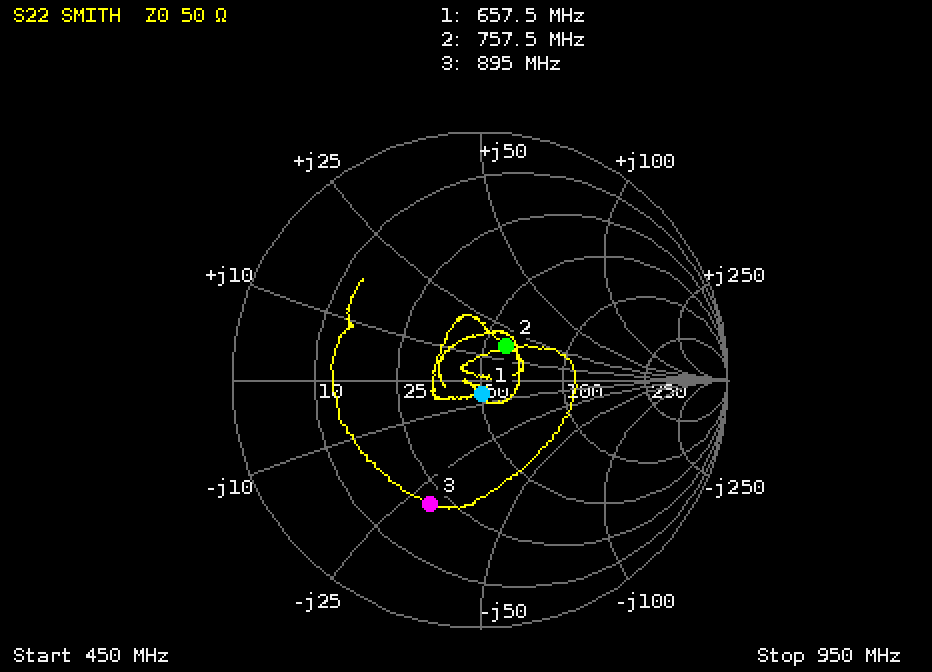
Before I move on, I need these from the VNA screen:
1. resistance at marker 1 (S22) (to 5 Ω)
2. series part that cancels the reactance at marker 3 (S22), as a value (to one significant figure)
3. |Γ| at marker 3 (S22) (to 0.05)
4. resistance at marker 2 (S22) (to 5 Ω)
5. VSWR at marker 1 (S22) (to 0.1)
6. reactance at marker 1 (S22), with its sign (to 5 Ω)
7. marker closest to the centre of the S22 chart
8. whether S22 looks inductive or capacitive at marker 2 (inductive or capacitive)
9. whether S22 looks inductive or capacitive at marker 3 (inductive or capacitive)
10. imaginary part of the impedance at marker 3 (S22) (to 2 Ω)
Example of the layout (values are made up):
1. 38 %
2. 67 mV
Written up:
1. 50 Ω
2. 5 nH
3. 0.55
4. 60 Ω
5. 1.1
6. -5 Ω
7. marker 1
8. inductive
9. capacitive
10. -30 Ω
